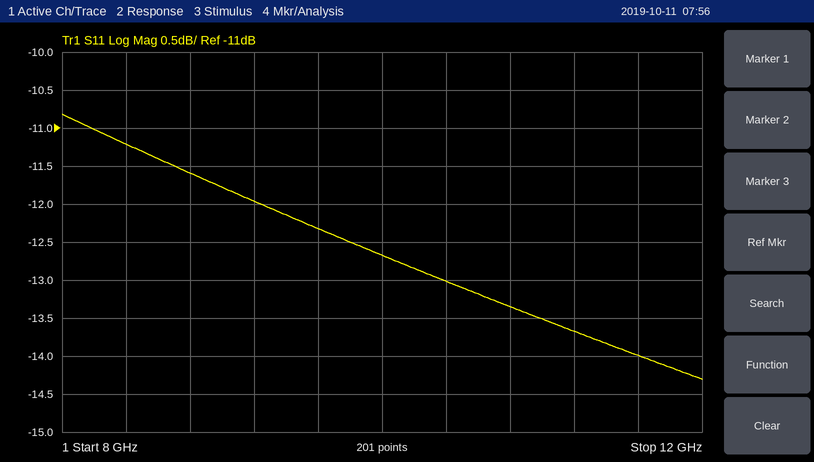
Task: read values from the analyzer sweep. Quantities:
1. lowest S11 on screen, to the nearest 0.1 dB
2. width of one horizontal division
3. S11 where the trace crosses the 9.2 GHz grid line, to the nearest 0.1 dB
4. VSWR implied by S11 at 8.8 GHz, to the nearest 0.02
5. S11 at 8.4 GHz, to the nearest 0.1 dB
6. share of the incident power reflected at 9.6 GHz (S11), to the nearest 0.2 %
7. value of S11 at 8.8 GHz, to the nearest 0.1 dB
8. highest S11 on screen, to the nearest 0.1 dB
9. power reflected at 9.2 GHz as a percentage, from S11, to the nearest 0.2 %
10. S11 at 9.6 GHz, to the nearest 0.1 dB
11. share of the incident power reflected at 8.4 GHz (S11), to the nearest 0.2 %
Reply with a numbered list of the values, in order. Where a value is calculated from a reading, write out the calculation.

1. -14.3 dB
2. 400 MHz
3. -12.0 dB
4. |Γ| = 10^(-11.6/20) = 0.2630; VSWR = (1 + 0.2630)/(1 − 0.2630) ≈ 1.71, so 1.72 to the nearest 0.02
5. -11.2 dB
6. 10^(-12.3/10) ≈ 5.89 %, so 5.8 % to the nearest 0.2 %
7. -11.6 dB
8. -10.8 dB
9. 10^(-12/10) ≈ 6.31 %, so 6.4 % to the nearest 0.2 %
10. -12.3 dB
11. 10^(-11.2/10) ≈ 7.6 %
